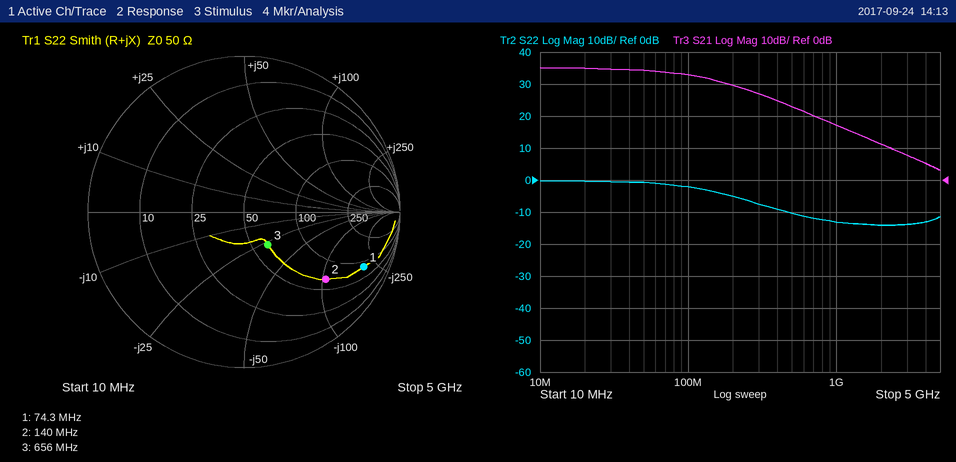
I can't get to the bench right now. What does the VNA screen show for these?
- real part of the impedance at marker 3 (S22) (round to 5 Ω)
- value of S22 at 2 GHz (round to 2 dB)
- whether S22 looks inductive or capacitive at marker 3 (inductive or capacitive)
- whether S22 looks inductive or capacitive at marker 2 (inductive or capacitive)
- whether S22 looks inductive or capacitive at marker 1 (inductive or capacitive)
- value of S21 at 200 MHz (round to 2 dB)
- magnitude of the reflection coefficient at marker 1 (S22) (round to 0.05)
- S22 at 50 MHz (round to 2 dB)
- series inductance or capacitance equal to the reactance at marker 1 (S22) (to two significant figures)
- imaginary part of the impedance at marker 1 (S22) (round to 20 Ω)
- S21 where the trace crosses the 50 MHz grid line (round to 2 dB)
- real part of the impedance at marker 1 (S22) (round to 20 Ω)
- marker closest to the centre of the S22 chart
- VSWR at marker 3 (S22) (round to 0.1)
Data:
60 Ω
-14 dB
capacitive
capacitive
capacitive
30 dB
0.85
0 dB
11 pF
-200 Ω
34 dB
80 Ω
marker 3
1.7
